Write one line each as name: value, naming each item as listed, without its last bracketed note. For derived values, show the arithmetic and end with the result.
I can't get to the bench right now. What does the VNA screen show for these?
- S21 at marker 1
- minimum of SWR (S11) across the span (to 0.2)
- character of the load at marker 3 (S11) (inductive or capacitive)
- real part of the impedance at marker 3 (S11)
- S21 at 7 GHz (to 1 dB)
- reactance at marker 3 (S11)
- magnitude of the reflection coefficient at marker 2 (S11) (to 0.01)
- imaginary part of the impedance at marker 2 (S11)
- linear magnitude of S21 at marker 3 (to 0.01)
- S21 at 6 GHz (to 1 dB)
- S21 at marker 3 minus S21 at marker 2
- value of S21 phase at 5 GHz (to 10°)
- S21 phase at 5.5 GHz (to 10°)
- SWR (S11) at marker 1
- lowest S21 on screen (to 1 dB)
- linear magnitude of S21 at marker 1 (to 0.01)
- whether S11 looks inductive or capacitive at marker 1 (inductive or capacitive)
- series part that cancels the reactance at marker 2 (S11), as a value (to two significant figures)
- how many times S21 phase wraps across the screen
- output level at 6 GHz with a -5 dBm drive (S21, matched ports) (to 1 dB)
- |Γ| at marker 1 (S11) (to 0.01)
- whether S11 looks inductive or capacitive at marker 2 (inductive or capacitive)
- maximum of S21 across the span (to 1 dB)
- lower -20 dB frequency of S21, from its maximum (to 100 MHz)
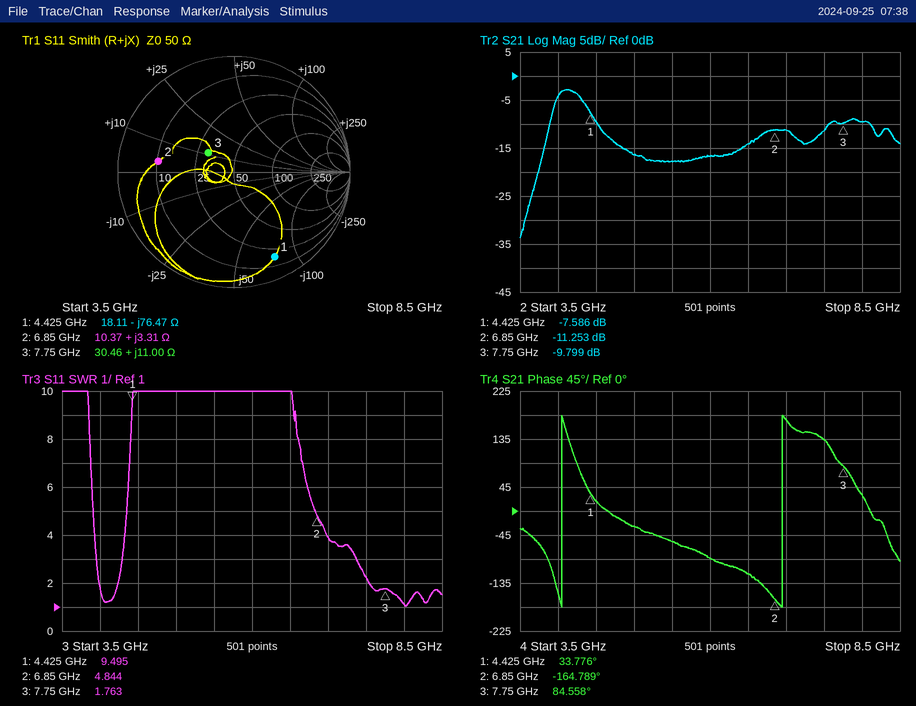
S21 at marker 1: -7.586 dB
minimum of SWR (S11) across the span: 1.0
character of the load at marker 3 (S11): inductive
real part of the impedance at marker 3: 30.46 Ω
S21 at 7 GHz: -11 dB
reactance at marker 3: +11.00 Ω
magnitude of the reflection coefficient at marker 2 (S11): 0.66
imaginary part of the impedance at marker 2: +3.31 Ω
linear magnitude of S21 at marker 3: 10^(-9.799/20) ≈ 0.32
S21 at 6 GHz: -17 dB
S21 at marker 3 minus S21 at marker 2: -9.799 − (-11.253) = 1.454 dB
value of S21 phase at 5 GHz: -30°
S21 phase at 5.5 GHz: -60°
SWR (S11) at marker 1: 9.495
lowest S21 on screen: -34 dB
linear magnitude of S21 at marker 1: 10^(-7.586/20) ≈ 0.42
whether S11 looks inductive or capacitive at marker 1: capacitive
series part that cancels the reactance at marker 2 (S11), as a value: C = 1/(2π × 6.85 GHz × 3.31 Ω) ≈ 7.0 pF
how many times S21 phase wraps across the screen: 2
output level at 6 GHz with a -5 dBm drive (S21, matched ports): -5 dBm + (-17 dB) = -22 dBm
|Γ| at marker 1 (S11): 0.81
whether S11 looks inductive or capacitive at marker 2: inductive
maximum of S21 across the span: -3 dB
lower -20 dB frequency of S21, from its maximum: 3.7 GHz
